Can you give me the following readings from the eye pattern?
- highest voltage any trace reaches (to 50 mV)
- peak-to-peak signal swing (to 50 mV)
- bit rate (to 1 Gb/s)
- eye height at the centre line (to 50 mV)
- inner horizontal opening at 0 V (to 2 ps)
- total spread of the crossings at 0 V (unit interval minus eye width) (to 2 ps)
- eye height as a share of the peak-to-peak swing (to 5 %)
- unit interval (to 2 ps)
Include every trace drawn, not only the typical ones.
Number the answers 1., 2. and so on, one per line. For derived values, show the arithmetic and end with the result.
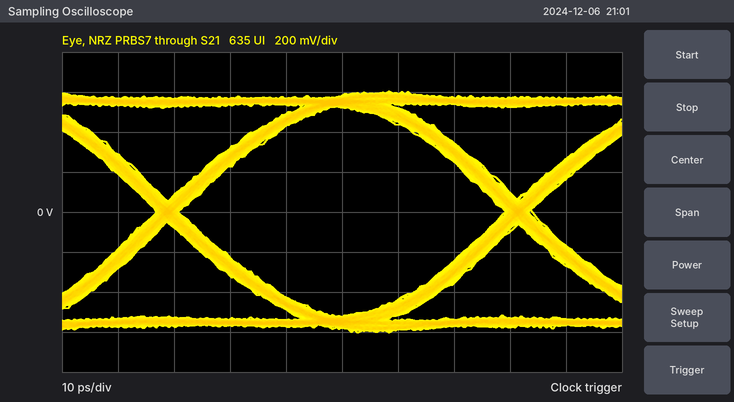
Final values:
1. 600 mV
2. 1.20 V
3. 16 Gb/s
4. 1.05 V
5. 58 ps
6. 4 ps
7. 1.05 V / 1.20 V ≈ 87.5 %, so 85 % to the nearest 5 %
8. 62 ps
